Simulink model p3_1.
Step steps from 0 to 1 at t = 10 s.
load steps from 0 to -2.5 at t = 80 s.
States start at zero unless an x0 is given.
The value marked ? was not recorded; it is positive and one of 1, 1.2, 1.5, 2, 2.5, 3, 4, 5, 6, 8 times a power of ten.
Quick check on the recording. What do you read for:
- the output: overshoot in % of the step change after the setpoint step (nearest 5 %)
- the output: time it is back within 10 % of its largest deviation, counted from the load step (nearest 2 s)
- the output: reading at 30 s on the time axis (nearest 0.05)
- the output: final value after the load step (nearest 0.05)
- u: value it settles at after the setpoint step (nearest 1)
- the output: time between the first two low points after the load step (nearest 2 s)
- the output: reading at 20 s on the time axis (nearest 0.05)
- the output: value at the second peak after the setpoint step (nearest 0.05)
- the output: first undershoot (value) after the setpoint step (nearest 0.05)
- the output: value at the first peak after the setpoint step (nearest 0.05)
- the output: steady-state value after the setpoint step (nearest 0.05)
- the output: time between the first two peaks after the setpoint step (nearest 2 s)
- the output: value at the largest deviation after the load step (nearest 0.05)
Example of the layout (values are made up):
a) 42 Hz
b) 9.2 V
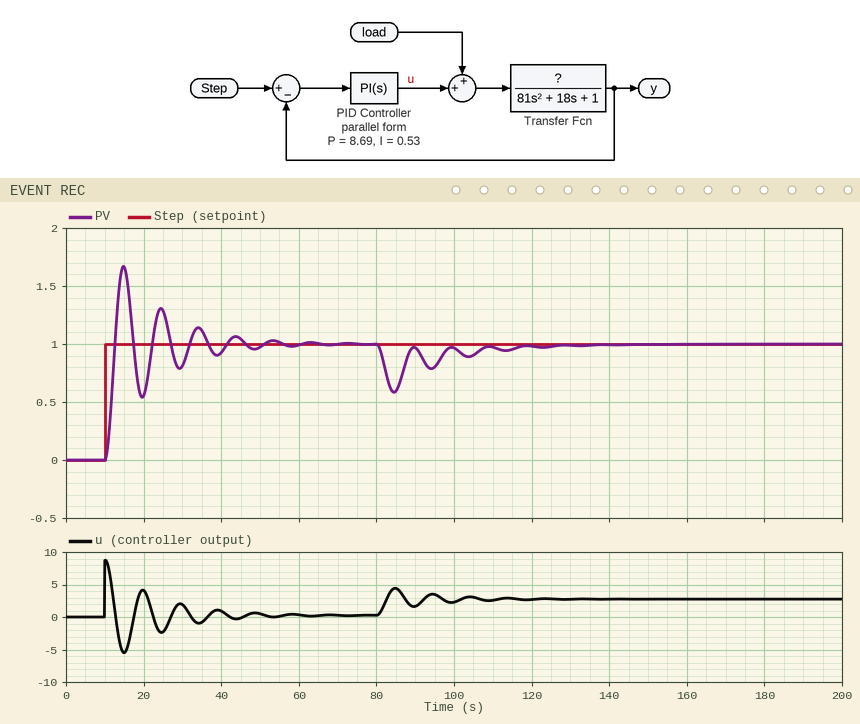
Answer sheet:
a) 65 %
b) 36 s
c) 0.80
d) 1.00
e) 0
f) 10 s
g) 0.55
h) 1.30
i) 0.55
j) 1.65
k) 1.00
l) 10 s
m) 0.60
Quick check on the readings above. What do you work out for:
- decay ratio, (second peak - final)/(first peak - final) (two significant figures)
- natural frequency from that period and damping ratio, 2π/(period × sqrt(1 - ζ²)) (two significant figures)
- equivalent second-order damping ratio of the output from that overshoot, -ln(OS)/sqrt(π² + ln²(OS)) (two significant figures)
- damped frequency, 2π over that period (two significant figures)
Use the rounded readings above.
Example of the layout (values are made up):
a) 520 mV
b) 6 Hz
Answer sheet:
a) 0.46
b) 0.63 rad/s
c) 0.14
d) 0.63 rad/s
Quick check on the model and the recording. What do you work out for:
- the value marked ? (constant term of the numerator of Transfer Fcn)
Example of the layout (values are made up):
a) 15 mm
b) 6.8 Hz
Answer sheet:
a) 4
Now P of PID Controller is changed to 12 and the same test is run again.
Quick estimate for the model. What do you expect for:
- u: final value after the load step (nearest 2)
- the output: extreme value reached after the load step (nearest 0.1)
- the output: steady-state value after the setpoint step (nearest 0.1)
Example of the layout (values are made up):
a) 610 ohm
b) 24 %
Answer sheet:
a) 2
b) 0.7
c) 1.0
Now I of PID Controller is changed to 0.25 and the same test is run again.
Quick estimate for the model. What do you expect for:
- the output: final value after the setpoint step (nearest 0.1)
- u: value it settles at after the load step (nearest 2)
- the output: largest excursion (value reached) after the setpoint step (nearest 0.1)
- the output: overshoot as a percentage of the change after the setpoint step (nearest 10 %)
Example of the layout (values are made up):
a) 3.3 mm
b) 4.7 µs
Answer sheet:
a) 1.0
b) 2
c) 1.6
d) 60 %
